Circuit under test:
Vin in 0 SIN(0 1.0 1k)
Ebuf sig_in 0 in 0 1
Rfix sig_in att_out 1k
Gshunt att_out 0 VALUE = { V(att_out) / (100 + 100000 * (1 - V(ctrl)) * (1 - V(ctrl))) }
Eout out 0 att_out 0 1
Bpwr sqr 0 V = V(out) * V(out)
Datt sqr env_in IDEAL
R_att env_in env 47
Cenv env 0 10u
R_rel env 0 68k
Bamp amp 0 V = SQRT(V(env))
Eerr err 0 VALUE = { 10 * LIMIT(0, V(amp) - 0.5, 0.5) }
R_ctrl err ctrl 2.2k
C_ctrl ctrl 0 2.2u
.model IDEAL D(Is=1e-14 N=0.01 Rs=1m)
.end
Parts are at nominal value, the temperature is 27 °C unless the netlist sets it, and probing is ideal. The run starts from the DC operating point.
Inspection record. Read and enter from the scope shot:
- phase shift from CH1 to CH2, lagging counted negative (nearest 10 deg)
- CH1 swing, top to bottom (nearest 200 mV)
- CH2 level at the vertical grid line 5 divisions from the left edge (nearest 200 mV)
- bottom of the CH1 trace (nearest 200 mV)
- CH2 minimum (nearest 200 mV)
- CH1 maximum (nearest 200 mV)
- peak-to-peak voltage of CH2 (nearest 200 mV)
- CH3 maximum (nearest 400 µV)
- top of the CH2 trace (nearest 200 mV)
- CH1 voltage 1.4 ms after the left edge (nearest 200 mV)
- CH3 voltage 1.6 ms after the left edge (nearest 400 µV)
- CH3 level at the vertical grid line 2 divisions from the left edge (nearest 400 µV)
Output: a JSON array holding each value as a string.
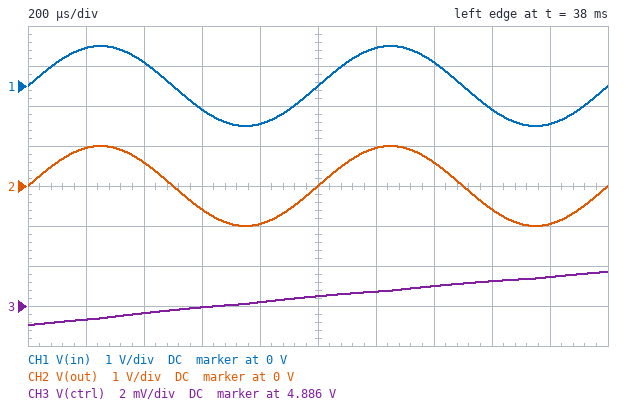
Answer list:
["0 deg", "2.0 V", "0 V", "-1.0 V", "-1.0 V", "1.0 V", "2.0 V", "4.8876 V", "1.0 V", "600 mV", "4.8872 V", "4.8856 V"]
